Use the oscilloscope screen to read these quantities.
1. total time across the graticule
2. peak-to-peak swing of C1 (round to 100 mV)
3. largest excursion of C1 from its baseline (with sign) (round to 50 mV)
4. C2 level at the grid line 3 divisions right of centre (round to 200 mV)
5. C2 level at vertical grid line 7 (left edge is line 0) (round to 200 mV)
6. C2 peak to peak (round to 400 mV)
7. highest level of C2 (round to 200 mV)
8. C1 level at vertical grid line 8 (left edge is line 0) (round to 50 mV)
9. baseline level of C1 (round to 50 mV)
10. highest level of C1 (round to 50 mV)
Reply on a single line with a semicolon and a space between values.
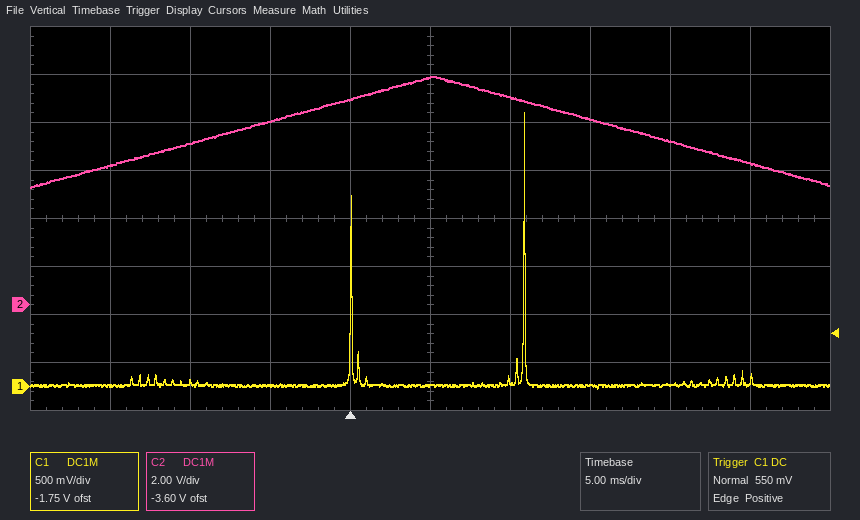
50 ms; 2.90 V; +2.85 V; 6.8 V; 7.8 V; 4.8 V; 9.6 V; 0 mV; 0 mV; 2.85 V
